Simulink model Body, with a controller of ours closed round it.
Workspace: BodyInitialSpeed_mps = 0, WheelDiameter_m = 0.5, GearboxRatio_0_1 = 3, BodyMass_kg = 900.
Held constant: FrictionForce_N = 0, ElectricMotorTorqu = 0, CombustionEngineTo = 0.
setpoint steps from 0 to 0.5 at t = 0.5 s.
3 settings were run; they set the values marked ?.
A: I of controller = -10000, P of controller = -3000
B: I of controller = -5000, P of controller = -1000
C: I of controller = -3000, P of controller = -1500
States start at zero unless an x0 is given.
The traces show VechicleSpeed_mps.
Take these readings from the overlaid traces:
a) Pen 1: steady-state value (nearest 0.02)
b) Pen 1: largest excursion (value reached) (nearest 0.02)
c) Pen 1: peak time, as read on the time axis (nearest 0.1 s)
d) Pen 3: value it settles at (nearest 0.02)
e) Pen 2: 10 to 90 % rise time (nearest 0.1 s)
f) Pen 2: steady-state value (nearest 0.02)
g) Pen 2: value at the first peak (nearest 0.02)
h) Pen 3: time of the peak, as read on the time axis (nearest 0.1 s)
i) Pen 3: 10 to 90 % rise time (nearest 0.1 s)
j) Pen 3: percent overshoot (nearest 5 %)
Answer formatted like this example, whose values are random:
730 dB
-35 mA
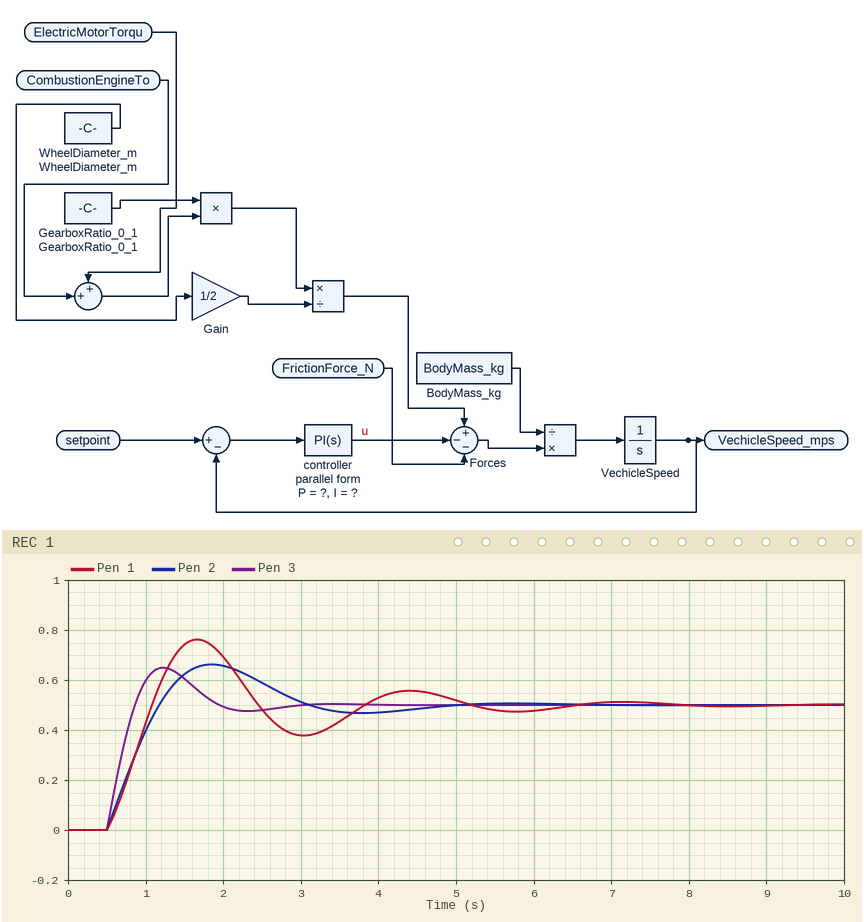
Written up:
0.50
0.76
1.7 s
0.50
0.5 s
0.50
0.66
1.2 s
0.3 s
30 %
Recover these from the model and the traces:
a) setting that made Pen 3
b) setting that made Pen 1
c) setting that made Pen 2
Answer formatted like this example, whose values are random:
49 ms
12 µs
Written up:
A
B
C
